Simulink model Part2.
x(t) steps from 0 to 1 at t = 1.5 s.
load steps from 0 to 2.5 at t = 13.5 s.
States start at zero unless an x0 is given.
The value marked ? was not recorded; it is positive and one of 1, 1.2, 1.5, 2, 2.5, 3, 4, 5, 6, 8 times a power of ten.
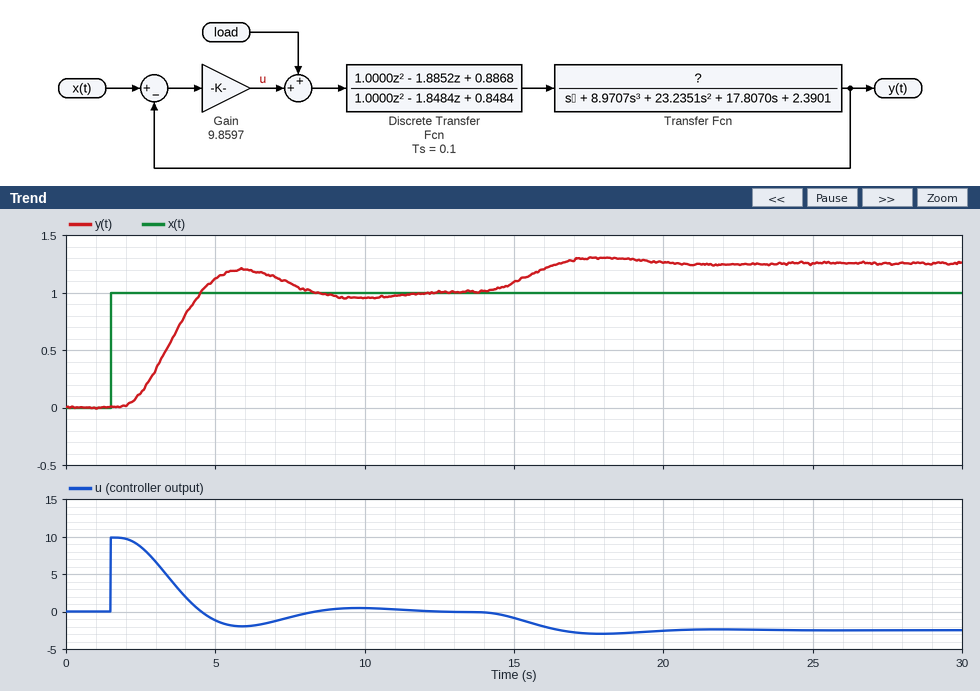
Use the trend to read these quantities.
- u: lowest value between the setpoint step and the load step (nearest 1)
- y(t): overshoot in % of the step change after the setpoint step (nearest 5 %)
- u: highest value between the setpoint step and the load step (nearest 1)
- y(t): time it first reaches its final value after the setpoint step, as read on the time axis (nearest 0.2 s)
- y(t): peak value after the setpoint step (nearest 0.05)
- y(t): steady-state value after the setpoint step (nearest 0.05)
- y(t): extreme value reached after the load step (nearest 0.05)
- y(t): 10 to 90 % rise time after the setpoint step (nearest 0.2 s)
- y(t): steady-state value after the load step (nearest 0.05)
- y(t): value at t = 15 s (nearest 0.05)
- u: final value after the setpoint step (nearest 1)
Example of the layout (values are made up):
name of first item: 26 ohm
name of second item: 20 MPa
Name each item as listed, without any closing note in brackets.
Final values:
u: lowest value between the setpoint step and the load step: -2
y(t): overshoot in % of the step change after the setpoint step: 20 %
u: highest value between the setpoint step and the load step: 10
y(t): time it first reaches its final value after the setpoint step, as read on the time axis: 4.6 s
y(t): peak value after the setpoint step: 1.20
y(t): steady-state value after the setpoint step: 1.00
y(t): extreme value reached after the load step: 1.30
y(t): 10 to 90 % rise time after the setpoint step: 1.8 s
y(t): steady-state value after the load step: 1.25
y(t): value at t = 15 s: 1.10
u: final value after the setpoint step: 0
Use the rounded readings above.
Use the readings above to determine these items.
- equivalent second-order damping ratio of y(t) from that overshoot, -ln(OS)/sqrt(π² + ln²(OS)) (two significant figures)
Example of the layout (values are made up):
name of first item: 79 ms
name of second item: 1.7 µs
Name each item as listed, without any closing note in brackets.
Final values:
equivalent second-order damping ratio of y(t) from that overshoot, -ln(OS)/sqrt(π² + ln²(OS)): 0.46
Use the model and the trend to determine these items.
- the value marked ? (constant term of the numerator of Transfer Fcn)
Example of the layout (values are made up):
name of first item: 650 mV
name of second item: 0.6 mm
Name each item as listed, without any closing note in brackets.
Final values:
the value marked ?: 1.5
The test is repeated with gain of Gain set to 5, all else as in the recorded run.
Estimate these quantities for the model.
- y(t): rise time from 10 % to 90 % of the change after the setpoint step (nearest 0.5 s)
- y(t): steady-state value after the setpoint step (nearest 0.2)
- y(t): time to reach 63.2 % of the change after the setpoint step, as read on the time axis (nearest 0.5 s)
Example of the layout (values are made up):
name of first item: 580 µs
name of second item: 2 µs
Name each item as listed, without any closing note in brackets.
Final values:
y(t): rise time from 10 % to 90 % of the change after the setpoint step: 4.0 s
y(t): steady-state value after the setpoint step: 1.0
y(t): time to reach 63.2 % of the change after the setpoint step, as read on the time axis: 5.0 s
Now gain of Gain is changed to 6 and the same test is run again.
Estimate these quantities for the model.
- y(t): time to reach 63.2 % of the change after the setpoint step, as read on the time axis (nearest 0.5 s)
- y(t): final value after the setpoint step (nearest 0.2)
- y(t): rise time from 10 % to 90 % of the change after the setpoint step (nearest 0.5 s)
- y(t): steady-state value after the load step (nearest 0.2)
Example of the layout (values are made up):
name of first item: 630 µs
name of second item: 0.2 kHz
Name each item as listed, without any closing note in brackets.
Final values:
y(t): time to reach 63.2 % of the change after the setpoint step, as read on the time axis: 4.5 s
y(t): final value after the setpoint step: 1.0
y(t): rise time from 10 % to 90 % of the change after the setpoint step: 3.0 s
y(t): steady-state value after the load step: 1.4
